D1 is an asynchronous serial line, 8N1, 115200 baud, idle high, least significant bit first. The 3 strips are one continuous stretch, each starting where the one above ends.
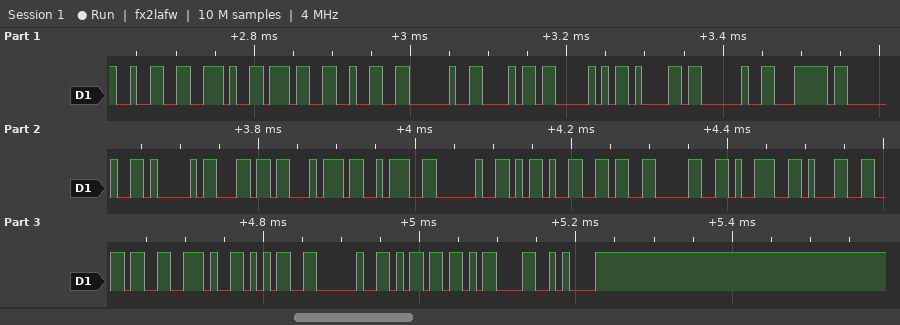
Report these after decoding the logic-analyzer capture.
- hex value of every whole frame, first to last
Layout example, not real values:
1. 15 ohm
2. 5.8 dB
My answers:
1. 32 2E 37 32 20 68 50 61 20 7C 20 41 6C 74 3A 20 2D 36 30 39 31 36 2E 35 20 6D 0D 0A
